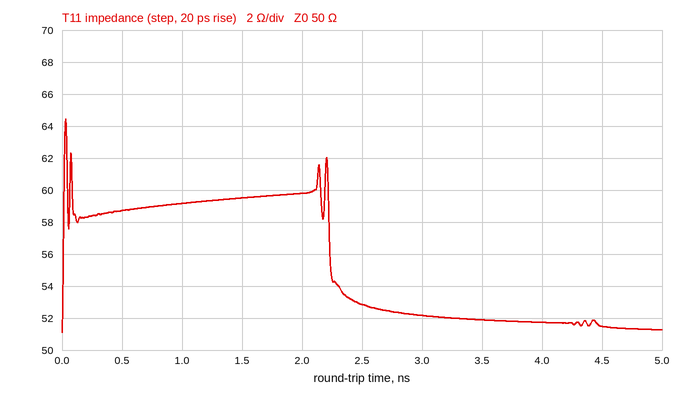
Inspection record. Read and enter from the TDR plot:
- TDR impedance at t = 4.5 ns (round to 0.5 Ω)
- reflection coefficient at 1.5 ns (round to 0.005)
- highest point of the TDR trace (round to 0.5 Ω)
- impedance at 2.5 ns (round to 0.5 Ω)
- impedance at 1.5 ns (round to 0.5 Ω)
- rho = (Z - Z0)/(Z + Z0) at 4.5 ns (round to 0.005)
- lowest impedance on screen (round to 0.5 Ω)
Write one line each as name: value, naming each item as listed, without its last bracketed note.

TDR impedance at t = 4.5 ns: 51.5 Ω
reflection coefficient at 1.5 ns: +0.085
highest point of the TDR trace: 64.5 Ω
impedance at 2.5 ns: 53.0 Ω
impedance at 1.5 ns: 59.5 Ω
rho = (Z - Z0)/(Z + Z0) at 4.5 ns: +0.015
lowest impedance on screen: 51.0 Ω
